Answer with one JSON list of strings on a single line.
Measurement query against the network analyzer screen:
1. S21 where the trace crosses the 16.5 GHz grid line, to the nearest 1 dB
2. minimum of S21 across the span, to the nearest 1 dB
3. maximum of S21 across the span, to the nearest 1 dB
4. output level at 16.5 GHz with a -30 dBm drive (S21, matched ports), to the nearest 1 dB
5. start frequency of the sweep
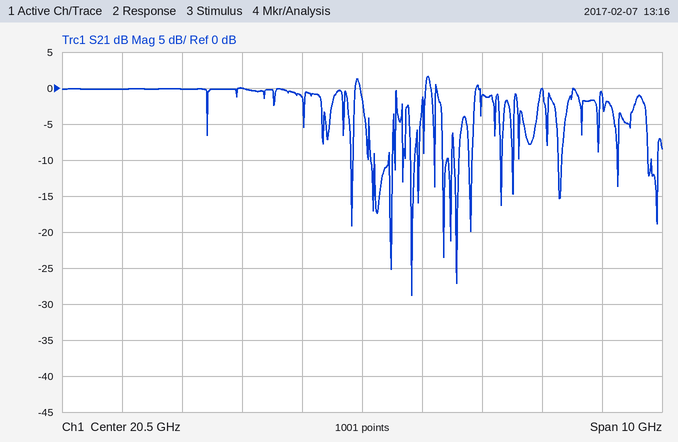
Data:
["0 dB", "-29 dB", "2 dB", "-30 dBm", "15.5 GHz"]
